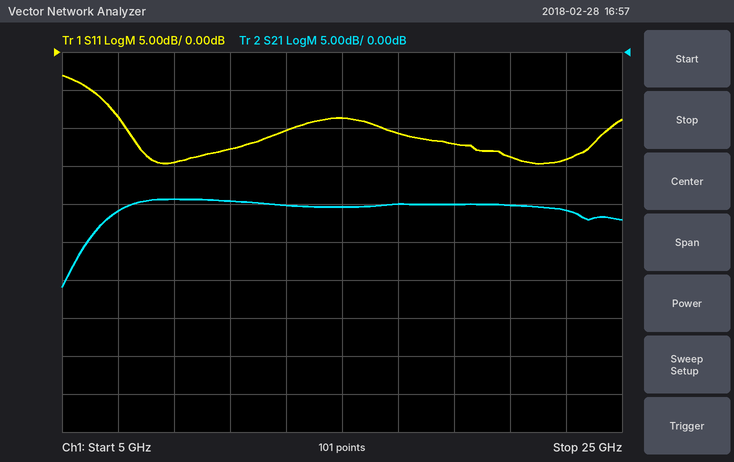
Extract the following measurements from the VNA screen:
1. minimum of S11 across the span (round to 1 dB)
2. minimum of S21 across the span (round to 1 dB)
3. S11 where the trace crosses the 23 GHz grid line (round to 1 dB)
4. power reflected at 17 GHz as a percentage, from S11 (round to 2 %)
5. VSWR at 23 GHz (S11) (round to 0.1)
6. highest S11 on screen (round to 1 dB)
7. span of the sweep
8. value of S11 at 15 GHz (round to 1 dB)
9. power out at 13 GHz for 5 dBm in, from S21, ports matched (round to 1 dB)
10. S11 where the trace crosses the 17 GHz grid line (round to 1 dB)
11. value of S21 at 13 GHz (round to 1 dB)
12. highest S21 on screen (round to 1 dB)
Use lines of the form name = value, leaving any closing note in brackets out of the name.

minimum of S11 across the span = -15 dB
minimum of S21 across the span = -31 dB
S11 where the trace crosses the 23 GHz grid line = -14 dB
power reflected at 17 GHz as a percentage, from S11 = 8 %
VSWR at 23 GHz (S11) = 1.5
highest S11 on screen = -3 dB
span of the sweep = 20 GHz
value of S11 at 15 GHz = -9 dB
power out at 13 GHz for 5 dBm in, from S21, ports matched = -15 dBm
S11 where the trace crosses the 17 GHz grid line = -11 dB
value of S21 at 13 GHz = -20 dB
highest S21 on screen = -19 dB
